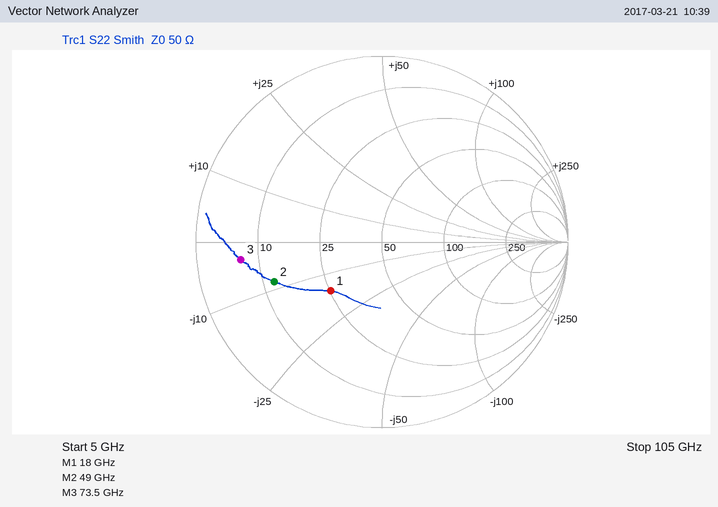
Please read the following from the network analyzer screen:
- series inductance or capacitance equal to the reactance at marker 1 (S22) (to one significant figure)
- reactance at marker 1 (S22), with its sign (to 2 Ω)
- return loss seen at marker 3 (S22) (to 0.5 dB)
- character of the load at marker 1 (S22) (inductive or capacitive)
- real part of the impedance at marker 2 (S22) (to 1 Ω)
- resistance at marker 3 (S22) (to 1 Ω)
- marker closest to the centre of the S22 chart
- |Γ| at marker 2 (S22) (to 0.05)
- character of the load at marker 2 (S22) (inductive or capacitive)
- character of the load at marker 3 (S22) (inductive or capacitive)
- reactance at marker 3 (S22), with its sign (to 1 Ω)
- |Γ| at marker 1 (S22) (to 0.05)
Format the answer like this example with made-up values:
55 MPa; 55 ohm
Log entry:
600 fF; -16 Ω; 2.5 dB; capacitive; 12 Ω; 7 Ω; marker 1; 0.60; capacitive; capacitive; -3 Ω; 0.40
